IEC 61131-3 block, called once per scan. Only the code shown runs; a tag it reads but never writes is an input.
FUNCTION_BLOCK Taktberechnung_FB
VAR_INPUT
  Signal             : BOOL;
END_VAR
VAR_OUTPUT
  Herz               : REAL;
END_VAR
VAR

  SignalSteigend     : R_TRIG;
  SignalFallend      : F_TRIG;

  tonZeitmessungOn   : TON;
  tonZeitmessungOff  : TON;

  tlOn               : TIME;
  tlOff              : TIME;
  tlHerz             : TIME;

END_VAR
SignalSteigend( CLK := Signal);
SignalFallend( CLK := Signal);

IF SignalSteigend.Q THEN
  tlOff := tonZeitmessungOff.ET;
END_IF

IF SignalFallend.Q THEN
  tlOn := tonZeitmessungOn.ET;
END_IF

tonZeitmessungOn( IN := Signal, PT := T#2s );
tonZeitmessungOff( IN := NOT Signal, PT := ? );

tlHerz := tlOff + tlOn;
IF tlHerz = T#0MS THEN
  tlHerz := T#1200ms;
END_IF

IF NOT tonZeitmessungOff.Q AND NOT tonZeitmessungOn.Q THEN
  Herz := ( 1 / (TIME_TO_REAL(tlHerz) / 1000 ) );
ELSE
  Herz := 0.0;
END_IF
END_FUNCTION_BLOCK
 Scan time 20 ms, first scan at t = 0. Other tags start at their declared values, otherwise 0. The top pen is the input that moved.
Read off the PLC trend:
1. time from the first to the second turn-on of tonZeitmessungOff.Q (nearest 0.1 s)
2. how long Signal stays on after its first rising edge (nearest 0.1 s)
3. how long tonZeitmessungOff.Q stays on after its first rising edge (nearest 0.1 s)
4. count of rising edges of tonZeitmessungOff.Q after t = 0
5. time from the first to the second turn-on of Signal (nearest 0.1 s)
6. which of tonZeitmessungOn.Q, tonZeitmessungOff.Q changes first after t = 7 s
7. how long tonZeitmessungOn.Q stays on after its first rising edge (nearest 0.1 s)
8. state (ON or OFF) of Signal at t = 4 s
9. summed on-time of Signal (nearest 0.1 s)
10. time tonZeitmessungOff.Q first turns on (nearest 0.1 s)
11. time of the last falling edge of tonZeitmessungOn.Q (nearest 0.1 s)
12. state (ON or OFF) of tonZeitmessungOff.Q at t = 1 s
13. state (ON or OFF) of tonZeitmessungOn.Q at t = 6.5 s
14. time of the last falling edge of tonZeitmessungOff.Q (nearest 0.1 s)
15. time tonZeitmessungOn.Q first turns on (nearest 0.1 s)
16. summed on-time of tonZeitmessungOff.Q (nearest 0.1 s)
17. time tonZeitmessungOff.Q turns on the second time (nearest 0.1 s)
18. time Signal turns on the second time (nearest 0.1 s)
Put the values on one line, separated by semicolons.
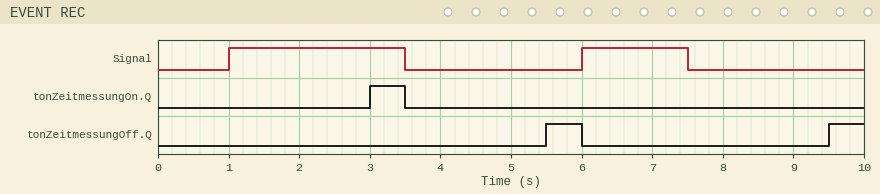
4.0 s; 2.5 s; 0.5 s; 2; 5.0 s; tonZeitmessungOff.Q; 0.5 s; OFF; 4.0 s; 5.5 s; 3.5 s; OFF; OFF; 6.0 s; 3.0 s; 1.0 s; 9.5 s; 6.0 s
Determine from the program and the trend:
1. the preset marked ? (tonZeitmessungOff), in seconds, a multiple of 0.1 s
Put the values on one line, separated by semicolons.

2.0 s
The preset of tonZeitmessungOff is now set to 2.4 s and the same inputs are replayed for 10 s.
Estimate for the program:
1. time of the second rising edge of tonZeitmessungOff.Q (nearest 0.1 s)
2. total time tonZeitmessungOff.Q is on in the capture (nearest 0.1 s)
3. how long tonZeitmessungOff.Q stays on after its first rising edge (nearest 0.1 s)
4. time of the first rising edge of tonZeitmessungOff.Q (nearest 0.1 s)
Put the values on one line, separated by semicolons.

9.9 s; 0.2 s; 0.1 s; 5.9 s
